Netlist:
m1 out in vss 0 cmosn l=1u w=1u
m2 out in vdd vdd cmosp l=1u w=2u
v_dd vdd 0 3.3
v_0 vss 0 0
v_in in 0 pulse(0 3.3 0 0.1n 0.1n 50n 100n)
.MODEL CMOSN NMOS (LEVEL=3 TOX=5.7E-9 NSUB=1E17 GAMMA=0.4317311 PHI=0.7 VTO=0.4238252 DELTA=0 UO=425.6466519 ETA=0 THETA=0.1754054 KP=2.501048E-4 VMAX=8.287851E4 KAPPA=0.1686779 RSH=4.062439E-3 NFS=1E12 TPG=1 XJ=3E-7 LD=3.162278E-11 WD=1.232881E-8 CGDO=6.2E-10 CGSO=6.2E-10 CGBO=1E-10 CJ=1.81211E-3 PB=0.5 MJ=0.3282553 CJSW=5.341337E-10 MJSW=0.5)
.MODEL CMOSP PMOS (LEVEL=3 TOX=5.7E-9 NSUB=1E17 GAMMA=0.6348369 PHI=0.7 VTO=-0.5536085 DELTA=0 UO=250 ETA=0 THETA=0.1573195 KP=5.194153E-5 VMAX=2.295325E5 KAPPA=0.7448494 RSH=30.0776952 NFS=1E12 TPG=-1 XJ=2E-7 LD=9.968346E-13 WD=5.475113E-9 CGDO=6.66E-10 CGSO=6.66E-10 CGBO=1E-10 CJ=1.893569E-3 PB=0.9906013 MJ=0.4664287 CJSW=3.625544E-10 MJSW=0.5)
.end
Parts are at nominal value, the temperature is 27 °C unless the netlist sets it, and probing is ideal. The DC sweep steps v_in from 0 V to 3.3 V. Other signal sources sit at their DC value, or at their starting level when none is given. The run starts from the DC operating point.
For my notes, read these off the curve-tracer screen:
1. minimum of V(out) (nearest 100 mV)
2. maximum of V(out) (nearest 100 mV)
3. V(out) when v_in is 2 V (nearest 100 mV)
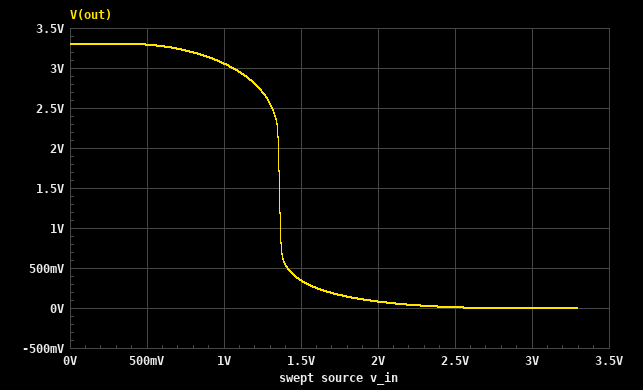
0 V
3.3 V
100 mV
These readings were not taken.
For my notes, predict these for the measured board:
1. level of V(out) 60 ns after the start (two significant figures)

3.3 V
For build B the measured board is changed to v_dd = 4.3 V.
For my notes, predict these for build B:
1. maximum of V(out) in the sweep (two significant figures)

4.3 V
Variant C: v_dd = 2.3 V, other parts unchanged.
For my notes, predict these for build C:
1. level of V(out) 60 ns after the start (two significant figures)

2.3 V
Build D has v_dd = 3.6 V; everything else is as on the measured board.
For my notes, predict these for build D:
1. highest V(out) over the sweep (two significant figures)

3.6 V
